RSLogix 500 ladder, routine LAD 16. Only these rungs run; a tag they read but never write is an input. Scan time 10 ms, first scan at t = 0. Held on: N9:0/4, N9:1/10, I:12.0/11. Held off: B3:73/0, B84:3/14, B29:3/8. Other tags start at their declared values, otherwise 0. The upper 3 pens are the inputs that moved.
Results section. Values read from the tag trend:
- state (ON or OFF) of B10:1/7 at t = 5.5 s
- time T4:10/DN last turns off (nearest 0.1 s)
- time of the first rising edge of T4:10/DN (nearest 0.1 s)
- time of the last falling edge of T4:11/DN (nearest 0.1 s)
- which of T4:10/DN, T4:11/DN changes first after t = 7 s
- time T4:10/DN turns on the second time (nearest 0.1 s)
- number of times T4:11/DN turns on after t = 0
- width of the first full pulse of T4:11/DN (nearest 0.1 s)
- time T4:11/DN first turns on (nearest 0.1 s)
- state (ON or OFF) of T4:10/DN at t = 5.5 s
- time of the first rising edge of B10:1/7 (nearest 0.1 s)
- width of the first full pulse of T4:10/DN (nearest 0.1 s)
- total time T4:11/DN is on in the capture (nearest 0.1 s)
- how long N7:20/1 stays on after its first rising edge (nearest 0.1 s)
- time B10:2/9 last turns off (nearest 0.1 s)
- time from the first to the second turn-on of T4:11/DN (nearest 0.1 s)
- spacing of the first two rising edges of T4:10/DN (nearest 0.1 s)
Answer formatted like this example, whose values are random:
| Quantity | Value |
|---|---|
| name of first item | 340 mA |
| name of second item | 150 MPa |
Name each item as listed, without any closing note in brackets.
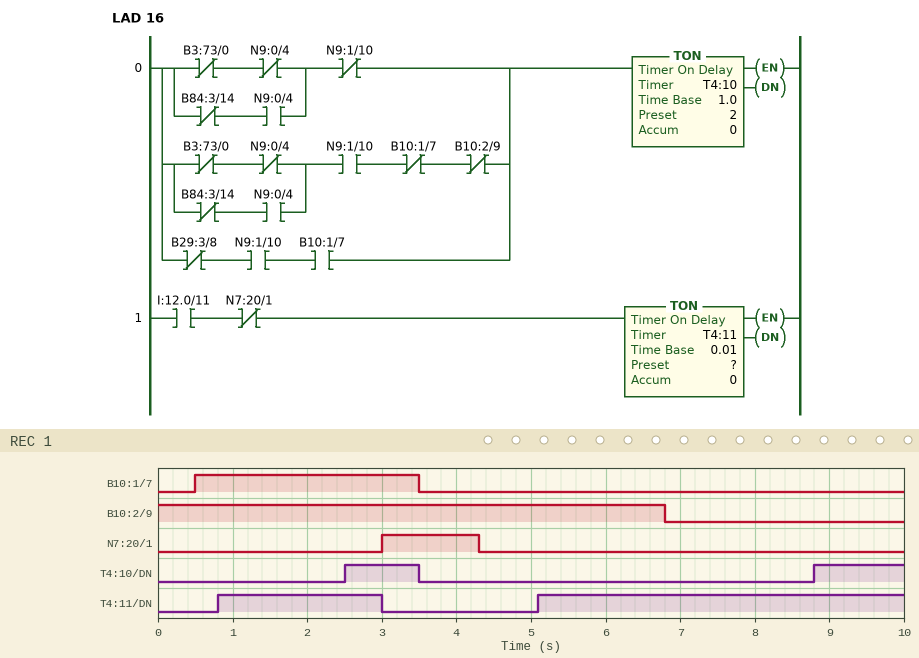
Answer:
| Quantity | Value |
|---|---|
| state (ON or OFF) of B10:1/7 at t = 5.5 s | OFF |
| time T4:10/DN last turns off | 3.5 s |
| time of the first rising edge of T4:10/DN | 2.5 s |
| time of the last falling edge of T4:11/DN | 3.0 s |
| which of T4:10/DN, T4:11/DN changes first after t = 7 s | T4:10/DN |
| time T4:10/DN turns on the second time | 8.8 s |
| number of times T4:11/DN turns on after t = 0 | 2 |
| width of the first full pulse of T4:11/DN | 2.2 s |
| time T4:11/DN first turns on | 0.8 s |
| state (ON or OFF) of T4:10/DN at t = 5.5 s | OFF |
| time of the first rising edge of B10:1/7 | 0.5 s |
| width of the first full pulse of T4:10/DN | 1.0 s |
| total time T4:11/DN is on in the capture | 7.1 s |
| how long N7:20/1 stays on after its first rising edge | 1.3 s |
| time B10:2/9 last turns off | 6.8 s |
| time from the first to the second turn-on of T4:11/DN | 4.3 s |
| spacing of the first two rising edges of T4:10/DN | 6.3 s |
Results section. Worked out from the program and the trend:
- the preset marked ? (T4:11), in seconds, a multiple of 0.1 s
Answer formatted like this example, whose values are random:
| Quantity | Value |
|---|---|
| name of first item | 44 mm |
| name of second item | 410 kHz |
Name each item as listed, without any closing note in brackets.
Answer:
| Quantity | Value |
|---|---|
| the preset marked ? (T4:11), in seconds, a multiple of 0.1 s | 0.8 s |
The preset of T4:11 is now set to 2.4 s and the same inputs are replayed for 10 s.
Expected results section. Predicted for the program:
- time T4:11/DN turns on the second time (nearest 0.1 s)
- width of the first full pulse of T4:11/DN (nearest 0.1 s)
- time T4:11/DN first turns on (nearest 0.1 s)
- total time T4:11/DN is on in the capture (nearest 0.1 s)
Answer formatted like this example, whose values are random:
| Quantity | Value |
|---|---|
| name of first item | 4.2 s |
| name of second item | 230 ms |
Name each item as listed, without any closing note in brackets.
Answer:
| Quantity | Value |
|---|---|
| time T4:11/DN turns on the second time | 6.7 s |
| width of the first full pulse of T4:11/DN | 0.6 s |
| time T4:11/DN first turns on | 2.4 s |
| total time T4:11/DN is on in the capture | 3.9 s |
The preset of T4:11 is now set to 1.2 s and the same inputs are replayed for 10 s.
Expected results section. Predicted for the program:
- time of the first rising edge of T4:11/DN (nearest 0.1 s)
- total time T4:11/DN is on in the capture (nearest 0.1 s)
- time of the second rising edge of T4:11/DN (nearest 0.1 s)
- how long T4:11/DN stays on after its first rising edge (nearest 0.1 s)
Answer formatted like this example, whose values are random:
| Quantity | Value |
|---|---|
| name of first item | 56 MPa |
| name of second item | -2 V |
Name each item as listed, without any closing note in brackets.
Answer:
| Quantity | Value |
|---|---|
| time of the first rising edge of T4:11/DN | 1.2 s |
| total time T4:11/DN is on in the capture | 6.3 s |
| time of the second rising edge of T4:11/DN | 5.5 s |
| how long T4:11/DN stays on after its first rising edge | 1.8 s |
